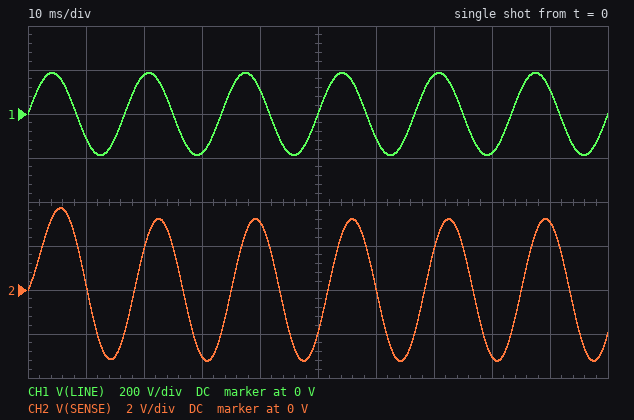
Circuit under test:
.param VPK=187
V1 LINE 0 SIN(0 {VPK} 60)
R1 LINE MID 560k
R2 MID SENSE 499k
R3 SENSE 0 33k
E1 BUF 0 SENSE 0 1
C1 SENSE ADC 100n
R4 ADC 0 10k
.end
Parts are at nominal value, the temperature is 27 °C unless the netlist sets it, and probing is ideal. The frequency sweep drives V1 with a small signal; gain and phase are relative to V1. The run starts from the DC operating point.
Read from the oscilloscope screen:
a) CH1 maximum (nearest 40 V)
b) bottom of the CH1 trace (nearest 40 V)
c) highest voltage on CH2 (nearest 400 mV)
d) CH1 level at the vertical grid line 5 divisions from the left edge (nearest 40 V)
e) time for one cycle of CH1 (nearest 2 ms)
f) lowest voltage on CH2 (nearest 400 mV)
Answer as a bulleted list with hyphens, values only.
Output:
- 200 V
- -200 V
- 3.6 V
- 0 V
- 16 ms
- -3.2 V
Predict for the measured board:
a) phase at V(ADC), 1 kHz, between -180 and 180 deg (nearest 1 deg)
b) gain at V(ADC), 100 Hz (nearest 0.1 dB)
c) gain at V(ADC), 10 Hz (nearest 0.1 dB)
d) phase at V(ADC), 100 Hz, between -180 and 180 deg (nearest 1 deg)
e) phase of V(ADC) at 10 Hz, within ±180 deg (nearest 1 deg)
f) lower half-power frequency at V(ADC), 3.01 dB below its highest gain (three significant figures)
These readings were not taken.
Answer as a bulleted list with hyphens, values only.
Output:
- 2 deg
- -43.4 dB
- -54.7 dB
- 21 deg
- 75 deg
- 37.9 Hz
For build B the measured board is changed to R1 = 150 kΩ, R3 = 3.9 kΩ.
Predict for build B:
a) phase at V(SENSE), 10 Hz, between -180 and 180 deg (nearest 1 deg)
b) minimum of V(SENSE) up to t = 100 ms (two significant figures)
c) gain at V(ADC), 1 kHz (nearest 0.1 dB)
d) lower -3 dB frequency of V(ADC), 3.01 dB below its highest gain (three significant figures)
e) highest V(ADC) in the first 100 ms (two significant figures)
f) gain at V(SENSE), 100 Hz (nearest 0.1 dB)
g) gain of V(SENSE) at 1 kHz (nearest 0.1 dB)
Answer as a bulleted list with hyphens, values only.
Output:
- -1 deg
- -1.1 V
- -47.4 dB
- 115 Hz
- 370 mV
- -45.5 dB
- -47.3 dB
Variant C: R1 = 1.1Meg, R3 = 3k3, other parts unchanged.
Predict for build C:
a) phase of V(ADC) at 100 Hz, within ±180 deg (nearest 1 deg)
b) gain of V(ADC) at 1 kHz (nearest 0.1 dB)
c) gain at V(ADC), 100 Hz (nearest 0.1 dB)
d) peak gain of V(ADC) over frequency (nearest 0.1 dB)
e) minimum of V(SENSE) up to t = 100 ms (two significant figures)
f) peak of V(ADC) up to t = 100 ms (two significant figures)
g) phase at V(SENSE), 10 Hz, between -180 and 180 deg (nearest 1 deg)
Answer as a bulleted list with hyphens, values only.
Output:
- 50 deg
- -56.3 dB
- -60.1 dB
- -56.2 dB
- -370 mV
- 130 mV
- -1 deg
